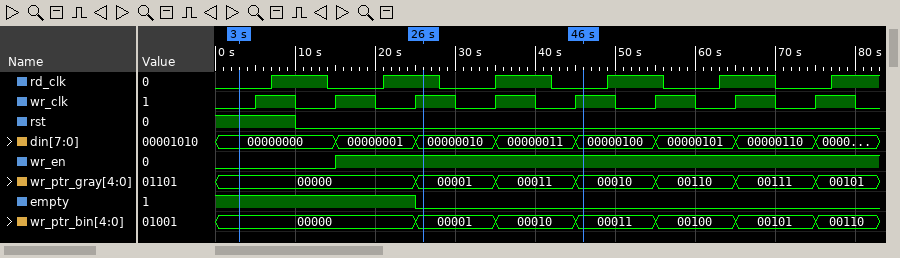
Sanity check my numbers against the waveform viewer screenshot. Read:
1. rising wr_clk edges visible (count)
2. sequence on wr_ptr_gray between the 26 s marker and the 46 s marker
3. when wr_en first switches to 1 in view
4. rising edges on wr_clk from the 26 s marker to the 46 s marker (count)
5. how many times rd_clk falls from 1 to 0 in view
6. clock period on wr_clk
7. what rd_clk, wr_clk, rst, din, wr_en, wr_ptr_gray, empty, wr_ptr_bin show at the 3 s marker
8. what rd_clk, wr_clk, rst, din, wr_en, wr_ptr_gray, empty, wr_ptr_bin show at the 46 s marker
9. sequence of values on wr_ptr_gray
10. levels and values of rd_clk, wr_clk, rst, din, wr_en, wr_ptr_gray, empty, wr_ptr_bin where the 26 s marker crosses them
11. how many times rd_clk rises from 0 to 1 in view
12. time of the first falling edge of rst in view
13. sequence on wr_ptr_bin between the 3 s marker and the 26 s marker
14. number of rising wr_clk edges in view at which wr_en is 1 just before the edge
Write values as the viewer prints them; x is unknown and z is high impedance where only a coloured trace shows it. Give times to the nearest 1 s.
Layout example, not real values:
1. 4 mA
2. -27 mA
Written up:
1. 8
2. 00001, 00011, 00010
3. 15 s
4. 2
5. 5
6. 10 s
7. rd_clk=0, wr_clk=0, rst=1, din=00000000, wr_en=0, wr_ptr_gray=00000, empty=1, wr_ptr_bin=00000
8. rd_clk=0, wr_clk=1, rst=0, din=00000100, wr_en=1, wr_ptr_gray=00010, empty=0, wr_ptr_bin=00011
9. 00000, 00001, 00011, 00010, 00110, 00111, 00101
10. rd_clk=1, wr_clk=1, rst=0, din=00000010, wr_en=1, wr_ptr_gray=00001, empty=0, wr_ptr_bin=00001
11. 6
12. 10 s
13. 00000, 00001
14. 6
